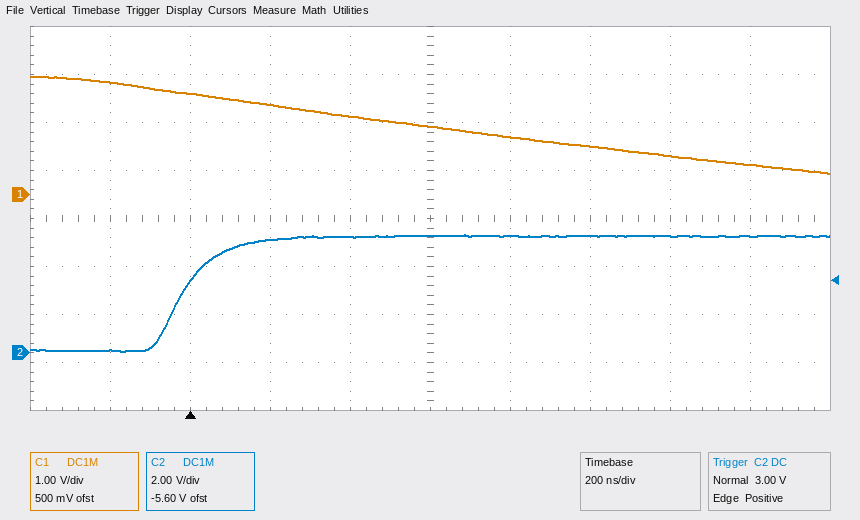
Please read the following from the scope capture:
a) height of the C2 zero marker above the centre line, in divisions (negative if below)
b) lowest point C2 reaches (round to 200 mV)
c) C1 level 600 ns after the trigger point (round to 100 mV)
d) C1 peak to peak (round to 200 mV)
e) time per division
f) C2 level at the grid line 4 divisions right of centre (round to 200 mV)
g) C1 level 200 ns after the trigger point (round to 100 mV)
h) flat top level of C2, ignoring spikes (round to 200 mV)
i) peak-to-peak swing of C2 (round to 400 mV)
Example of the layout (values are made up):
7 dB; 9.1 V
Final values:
-2.8 div; 0.0 V; 1.4 V; 2.0 V; 200 ns; 4.8 V; 1.9 V; 4.8 V; 4.8 V
